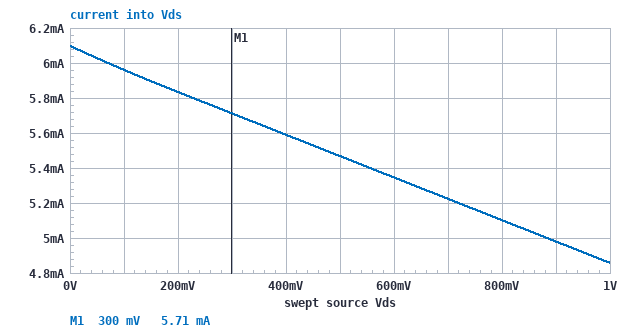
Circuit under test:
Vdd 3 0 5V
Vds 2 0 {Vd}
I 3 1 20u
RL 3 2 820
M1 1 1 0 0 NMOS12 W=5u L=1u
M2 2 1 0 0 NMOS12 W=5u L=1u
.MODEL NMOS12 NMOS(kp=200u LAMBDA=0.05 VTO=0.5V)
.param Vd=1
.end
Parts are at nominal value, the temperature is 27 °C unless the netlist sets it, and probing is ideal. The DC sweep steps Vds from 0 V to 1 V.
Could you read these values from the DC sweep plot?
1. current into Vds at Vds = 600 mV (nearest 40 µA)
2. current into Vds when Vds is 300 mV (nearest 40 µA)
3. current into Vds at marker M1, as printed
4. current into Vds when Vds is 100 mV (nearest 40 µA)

5.36 mA
5.72 mA
5.71 mA
5.96 mA
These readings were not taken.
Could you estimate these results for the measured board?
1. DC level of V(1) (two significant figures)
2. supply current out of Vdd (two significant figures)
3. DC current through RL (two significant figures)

700 mV
4.9 mA
4.9 mA
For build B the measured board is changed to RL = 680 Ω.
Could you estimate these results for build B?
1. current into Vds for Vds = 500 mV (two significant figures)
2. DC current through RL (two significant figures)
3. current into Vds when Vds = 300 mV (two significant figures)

6.6 mA
5.9 mA
6.9 mA
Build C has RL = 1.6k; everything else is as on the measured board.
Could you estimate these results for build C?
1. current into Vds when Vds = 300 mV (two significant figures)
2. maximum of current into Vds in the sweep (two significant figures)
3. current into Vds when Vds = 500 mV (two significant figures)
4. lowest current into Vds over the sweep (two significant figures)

2.9 mA
3.1 mA
2.8 mA
2.5 mA
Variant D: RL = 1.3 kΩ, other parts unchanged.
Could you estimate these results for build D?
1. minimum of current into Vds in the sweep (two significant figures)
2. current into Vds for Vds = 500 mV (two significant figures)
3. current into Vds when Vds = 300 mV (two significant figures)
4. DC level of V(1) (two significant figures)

3.1 mA
3.4 mA
3.6 mA
700 mV
